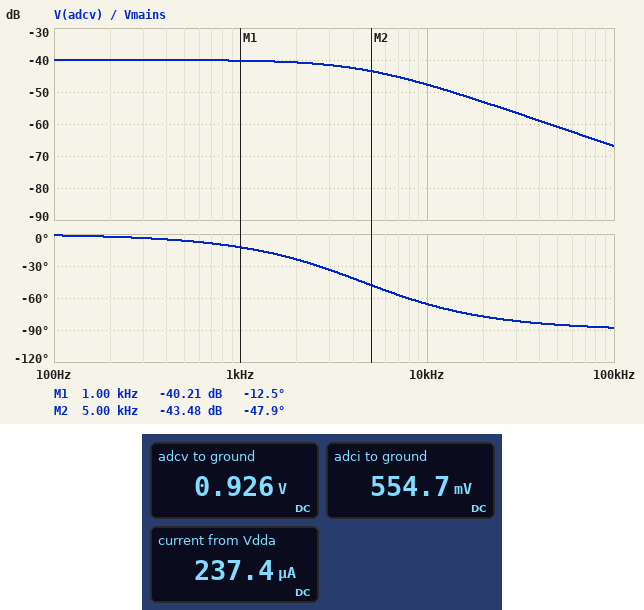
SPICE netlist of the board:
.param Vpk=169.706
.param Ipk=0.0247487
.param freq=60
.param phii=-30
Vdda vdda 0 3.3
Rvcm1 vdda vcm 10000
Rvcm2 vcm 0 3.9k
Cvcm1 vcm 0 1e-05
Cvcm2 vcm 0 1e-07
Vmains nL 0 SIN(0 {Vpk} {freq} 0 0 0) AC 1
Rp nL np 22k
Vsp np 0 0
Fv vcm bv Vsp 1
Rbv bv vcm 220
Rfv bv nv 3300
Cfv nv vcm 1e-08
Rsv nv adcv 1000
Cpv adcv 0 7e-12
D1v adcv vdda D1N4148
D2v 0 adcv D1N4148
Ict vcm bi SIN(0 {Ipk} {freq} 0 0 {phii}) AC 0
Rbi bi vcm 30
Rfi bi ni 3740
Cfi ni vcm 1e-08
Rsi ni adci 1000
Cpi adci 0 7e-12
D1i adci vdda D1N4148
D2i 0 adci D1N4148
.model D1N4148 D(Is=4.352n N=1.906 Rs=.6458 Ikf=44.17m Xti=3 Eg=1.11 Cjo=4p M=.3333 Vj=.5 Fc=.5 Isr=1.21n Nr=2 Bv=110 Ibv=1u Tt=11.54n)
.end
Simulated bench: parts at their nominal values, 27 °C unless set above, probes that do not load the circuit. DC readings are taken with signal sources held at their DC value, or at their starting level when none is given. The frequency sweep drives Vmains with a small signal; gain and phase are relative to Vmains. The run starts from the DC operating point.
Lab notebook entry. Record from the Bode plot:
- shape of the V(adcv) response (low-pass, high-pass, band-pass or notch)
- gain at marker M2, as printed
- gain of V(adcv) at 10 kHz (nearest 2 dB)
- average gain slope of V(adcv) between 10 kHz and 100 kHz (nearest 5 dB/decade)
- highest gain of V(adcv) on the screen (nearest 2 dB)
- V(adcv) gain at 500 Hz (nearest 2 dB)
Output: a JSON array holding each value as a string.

["low-pass", "-43.48 dB", "-48 dB", "-20 dB/decade", "-40 dB", "-40 dB"]
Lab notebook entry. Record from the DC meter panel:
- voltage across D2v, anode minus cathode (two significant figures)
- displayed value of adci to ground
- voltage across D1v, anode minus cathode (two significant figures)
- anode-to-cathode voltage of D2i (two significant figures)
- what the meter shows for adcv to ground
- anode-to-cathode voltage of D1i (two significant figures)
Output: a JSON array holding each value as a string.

["-930 mV", "554.7 mV", "-2.4 V", "-550 mV", "0.926 V", "-2.7 V"]
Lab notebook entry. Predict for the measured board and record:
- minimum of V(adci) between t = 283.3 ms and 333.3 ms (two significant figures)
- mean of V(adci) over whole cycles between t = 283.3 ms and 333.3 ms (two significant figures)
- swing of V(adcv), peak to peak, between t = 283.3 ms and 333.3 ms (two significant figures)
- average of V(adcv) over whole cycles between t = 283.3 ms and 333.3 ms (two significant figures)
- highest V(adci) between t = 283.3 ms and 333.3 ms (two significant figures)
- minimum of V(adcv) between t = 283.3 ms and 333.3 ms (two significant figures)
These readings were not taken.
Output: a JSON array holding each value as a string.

["210 mV", "950 mV", "3.1 V", "990 mV", "1.7 V", "-470 mV"]
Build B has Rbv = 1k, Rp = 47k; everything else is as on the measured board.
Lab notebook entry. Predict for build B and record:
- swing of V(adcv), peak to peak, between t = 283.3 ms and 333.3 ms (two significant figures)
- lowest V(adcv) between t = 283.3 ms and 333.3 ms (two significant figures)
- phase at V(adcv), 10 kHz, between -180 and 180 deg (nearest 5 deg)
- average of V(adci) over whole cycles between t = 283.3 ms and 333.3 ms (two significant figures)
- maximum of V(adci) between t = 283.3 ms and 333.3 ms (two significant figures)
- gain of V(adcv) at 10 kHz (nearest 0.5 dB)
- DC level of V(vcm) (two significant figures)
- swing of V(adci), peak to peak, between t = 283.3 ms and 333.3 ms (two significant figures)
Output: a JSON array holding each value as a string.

["4.4 V", "-560 mV", "-70 deg", "1.1 V", "1.8 V", "-42.5 dB", "930 mV", "1.4 V"]
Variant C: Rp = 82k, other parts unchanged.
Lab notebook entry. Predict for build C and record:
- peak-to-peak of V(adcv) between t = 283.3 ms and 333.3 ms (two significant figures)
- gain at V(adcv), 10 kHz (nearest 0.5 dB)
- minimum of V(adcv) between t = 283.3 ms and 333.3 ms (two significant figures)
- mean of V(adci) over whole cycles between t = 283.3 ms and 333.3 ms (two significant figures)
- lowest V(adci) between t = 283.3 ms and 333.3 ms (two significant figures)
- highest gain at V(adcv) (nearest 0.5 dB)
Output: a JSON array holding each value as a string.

["910 mV", "-59.0 dB", "470 mV", "930 mV", "180 mV", "-51.5 dB"]
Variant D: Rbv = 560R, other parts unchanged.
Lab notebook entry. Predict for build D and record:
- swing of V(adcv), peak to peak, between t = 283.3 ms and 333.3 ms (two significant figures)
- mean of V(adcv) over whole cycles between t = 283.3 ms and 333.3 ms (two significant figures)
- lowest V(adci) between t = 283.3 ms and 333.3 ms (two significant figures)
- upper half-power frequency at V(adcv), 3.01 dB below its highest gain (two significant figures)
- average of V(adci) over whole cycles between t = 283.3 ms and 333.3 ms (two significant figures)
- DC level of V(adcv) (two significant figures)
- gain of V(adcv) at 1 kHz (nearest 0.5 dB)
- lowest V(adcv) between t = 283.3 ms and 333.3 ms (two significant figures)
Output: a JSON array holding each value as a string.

["4.4 V", "1.5 V", "440 mV", "4.1 kHz", "1.1 V", "930 mV", "-32.0 dB", "-580 mV"]
